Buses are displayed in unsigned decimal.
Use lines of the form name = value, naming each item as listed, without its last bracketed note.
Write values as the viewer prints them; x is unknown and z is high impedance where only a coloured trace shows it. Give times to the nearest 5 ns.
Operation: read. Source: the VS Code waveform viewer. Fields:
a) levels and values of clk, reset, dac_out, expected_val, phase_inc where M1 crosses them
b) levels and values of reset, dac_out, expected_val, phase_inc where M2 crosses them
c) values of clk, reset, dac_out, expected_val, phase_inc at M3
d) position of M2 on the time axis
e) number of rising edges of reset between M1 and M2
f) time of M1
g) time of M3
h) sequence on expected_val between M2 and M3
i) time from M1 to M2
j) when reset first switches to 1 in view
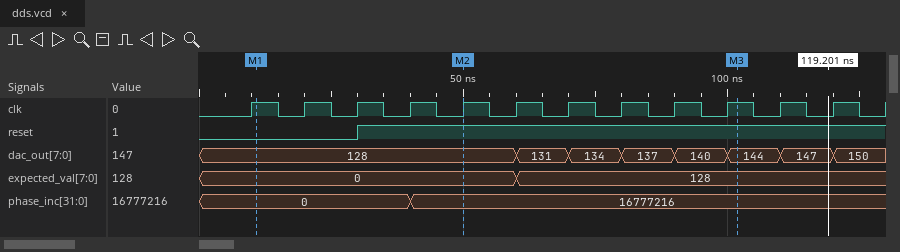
levels and values of clk, reset, dac_out, expected_val, phase_inc where M1 crosses them = clk=1, reset=0, dac_out=128, expected_val=0, phase_inc=0
levels and values of reset, dac_out, expected_val, phase_inc where M2 crosses them = reset=1, dac_out=128, expected_val=0, phase_inc=16777216
values of clk, reset, dac_out, expected_val, phase_inc at M3 = clk=1, reset=1, dac_out=144, expected_val=128, phase_inc=16777216
position of M2 on the time axis = 50 ns
number of rising edges of reset between M1 and M2 = 1
time of M1 = 10 ns
time of M3 = 100 ns
sequence on expected_val between M2 and M3 = 0, 128
time from M1 to M2 = 40 ns
when reset first switches to 1 in view = 30 ns
